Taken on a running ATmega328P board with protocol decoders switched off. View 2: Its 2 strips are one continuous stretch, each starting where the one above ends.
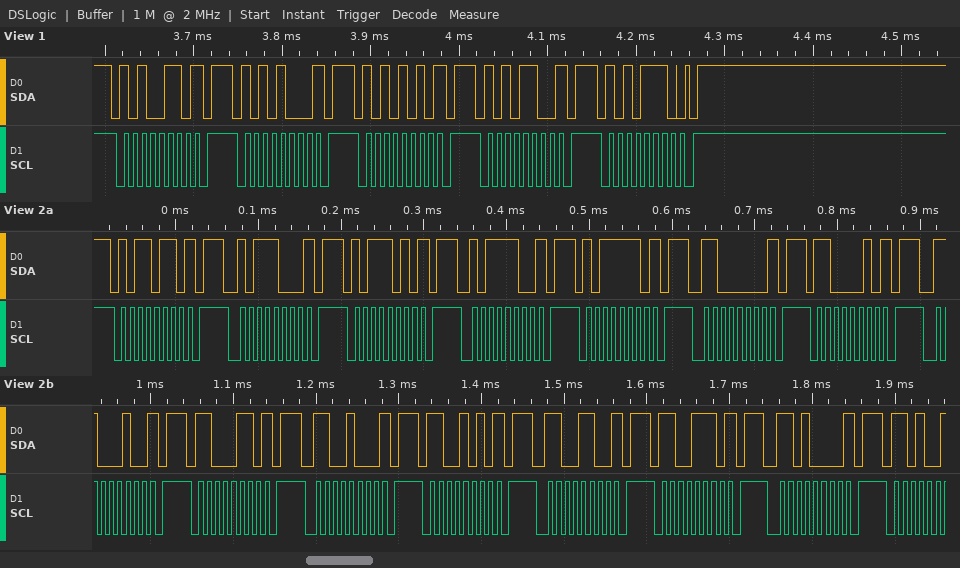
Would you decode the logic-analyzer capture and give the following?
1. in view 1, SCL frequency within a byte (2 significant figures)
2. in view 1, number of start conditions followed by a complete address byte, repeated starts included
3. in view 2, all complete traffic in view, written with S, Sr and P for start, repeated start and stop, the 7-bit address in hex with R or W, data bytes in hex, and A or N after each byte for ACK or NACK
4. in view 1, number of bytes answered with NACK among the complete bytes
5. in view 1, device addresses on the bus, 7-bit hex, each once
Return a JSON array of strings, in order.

["100 kHz", "5", "S 5BW N P S 5CW N P S 5DW N P S 5EW N P S 5FW N P S 60W N P S 61W N P S 62W N P S 63W N P S 64W N P S 65W N P S 66W N P S 67W N P S 68W N P", "4", "0x53 0x54 0x55 0x56 0x57"]
